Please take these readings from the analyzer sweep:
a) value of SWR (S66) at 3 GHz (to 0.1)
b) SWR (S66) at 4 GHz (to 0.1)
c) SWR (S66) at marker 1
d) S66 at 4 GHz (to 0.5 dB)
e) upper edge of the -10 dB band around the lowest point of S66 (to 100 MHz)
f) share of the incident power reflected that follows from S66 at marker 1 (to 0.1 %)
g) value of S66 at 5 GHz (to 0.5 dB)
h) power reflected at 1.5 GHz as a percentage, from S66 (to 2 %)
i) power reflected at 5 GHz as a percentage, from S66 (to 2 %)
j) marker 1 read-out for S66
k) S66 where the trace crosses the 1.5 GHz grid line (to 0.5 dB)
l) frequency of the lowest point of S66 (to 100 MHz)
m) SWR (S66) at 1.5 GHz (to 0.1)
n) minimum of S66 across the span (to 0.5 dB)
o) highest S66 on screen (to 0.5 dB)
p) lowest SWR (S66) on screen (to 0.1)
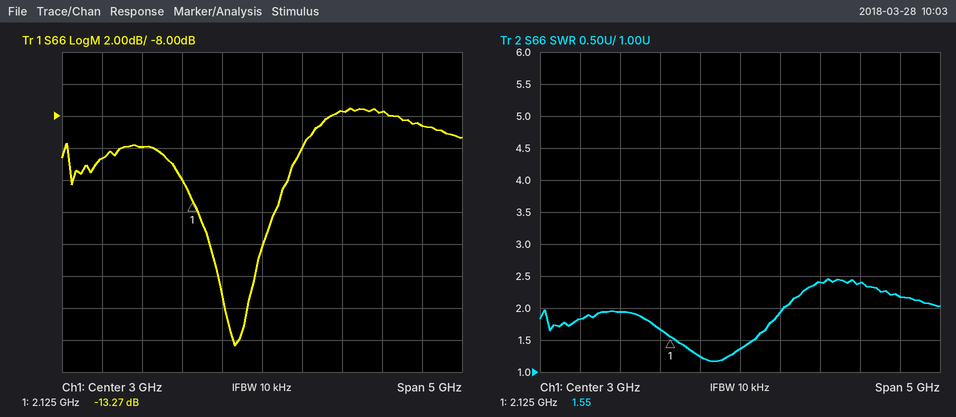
1.4
2.4
1.55
-7.5 dB
3.5 GHz
4.7 %
-8.5 dB
10 %
14 %
-13.27 dB
-10.0 dB
2.7 GHz
1.9
-22.5 dB
-7.5 dB
1.2
